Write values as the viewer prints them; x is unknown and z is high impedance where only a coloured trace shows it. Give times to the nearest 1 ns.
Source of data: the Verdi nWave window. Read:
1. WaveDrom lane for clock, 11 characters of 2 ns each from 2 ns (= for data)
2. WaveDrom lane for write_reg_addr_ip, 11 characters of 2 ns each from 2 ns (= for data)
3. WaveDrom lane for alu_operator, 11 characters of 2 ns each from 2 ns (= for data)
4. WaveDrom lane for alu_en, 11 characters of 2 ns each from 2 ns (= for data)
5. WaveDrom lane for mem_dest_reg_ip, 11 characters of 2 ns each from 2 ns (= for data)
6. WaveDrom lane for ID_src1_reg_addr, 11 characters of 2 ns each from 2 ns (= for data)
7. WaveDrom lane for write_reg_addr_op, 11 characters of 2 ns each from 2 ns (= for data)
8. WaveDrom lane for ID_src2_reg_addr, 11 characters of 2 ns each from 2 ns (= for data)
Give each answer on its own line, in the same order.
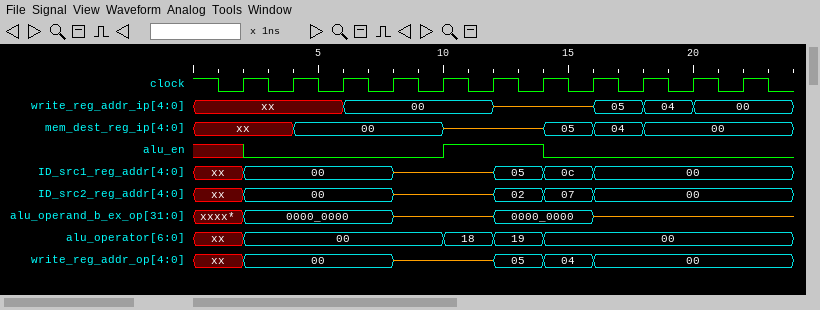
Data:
{name: 'clock', wave: 'p..........'}
{name: 'write_reg_addr_ip', wave: 'x.=..z.===.', data: '00 05 04 00'}
{name: 'alu_operator', wave: '=...===....', data: '00 18 19 00'}
{name: 'alu_en', wave: '0...1.0....'}
{name: 'mem_dest_reg_ip', wave: 'x=..z.===..', data: '00 05 04 00'}
{name: 'ID_src1_reg_addr', wave: '=..z.===...', data: '00 05 0c 00'}
{name: 'write_reg_addr_op', wave: '=..z.===...', data: '00 05 04 00'}
{name: 'ID_src2_reg_addr', wave: '=..z.===...', data: '00 02 07 00'}
